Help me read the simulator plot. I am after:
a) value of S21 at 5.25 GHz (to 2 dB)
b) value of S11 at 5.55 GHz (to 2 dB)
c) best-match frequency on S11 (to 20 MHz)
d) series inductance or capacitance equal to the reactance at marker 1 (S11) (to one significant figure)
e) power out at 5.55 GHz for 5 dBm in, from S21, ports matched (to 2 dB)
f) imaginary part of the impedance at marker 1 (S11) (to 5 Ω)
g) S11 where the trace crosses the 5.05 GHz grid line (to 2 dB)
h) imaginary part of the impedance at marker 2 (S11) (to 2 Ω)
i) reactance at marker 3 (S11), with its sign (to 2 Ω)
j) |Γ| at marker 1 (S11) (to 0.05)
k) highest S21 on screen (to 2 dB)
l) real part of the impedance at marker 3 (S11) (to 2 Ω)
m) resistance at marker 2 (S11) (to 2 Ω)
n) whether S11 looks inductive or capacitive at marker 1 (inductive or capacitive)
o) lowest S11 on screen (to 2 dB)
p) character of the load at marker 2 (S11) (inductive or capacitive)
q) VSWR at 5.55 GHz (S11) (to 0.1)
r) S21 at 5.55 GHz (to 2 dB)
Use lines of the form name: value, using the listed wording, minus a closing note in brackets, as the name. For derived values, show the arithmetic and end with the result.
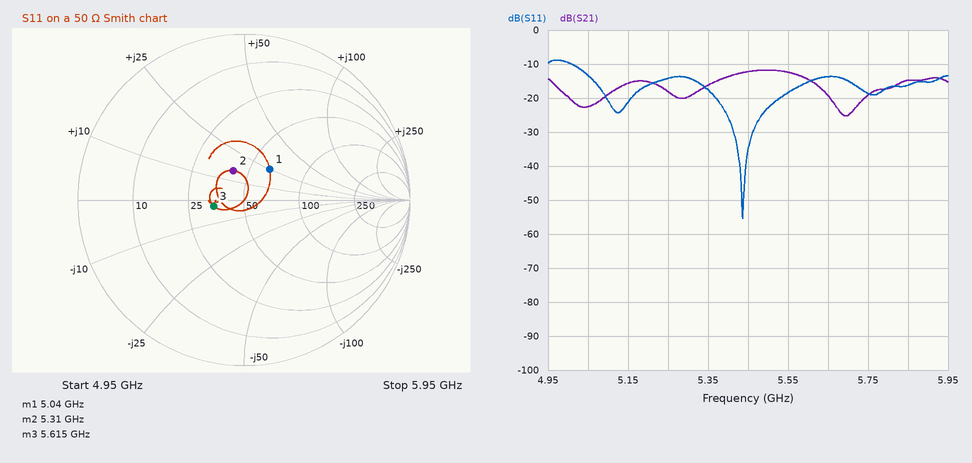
value of S21 at 5.25 GHz: -18 dB
value of S11 at 5.55 GHz: -18 dB
best-match frequency on S11: 5.44 GHz
series inductance or capacitance equal to the reactance at marker 1 (S11): L = 25 Ω/(2π × 5.04 GHz) ≈ 789 pH, so 800 pH to one significant figure
power out at 5.55 GHz for 5 dBm in, from S21, ports matched: 5 dBm + (-12 dB) = -8 dBm
imaginary part of the impedance at marker 1 (S11): +25 Ω
S11 where the trace crosses the 5.05 GHz grid line: -14 dB
imaginary part of the impedance at marker 2 (S11): +16 Ω
reactance at marker 3 (S11), with its sign: -2 Ω
|Γ| at marker 1 (S11): 0.25
highest S21 on screen: -12 dB
real part of the impedance at marker 3 (S11): 34 Ω
resistance at marker 2 (S11): 42 Ω
whether S11 looks inductive or capacitive at marker 1: inductive
lowest S11 on screen: -56 dB
character of the load at marker 2 (S11): inductive
VSWR at 5.55 GHz (S11): |Γ| = 10^(-18/20) = 0.1259; VSWR = (1 + 0.1259)/(1 − 0.1259) ≈ 1.3
S21 at 5.55 GHz: -12 dB
